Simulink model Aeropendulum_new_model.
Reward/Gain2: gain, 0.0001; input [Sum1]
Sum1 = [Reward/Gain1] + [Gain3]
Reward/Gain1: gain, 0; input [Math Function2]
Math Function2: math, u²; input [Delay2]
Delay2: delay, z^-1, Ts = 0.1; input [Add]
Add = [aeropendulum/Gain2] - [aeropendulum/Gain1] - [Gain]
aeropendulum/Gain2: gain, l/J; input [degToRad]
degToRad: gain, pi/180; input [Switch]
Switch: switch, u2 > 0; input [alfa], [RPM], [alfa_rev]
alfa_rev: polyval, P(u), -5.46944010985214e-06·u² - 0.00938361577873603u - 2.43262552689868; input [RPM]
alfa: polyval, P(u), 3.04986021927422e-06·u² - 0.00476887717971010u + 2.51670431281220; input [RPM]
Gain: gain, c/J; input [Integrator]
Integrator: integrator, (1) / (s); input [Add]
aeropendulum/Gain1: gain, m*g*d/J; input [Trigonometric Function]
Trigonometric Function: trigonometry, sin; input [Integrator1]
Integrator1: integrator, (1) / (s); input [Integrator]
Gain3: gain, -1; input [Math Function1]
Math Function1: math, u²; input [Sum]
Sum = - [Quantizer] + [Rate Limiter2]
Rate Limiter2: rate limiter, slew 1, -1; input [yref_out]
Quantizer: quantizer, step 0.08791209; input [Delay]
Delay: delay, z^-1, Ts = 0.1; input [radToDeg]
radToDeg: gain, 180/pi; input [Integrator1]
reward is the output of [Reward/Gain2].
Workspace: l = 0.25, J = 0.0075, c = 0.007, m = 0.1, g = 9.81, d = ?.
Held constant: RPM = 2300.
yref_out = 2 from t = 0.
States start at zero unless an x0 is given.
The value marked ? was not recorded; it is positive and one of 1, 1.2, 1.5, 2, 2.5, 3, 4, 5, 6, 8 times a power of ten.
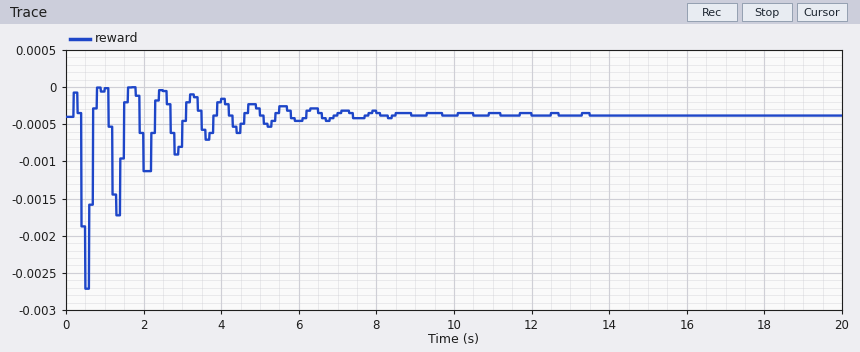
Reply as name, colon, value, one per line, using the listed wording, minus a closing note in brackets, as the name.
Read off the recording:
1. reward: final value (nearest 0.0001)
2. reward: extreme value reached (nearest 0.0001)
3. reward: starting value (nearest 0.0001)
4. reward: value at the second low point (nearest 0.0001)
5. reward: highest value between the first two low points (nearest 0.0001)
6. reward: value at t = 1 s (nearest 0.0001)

reward: final value: -0.0004
reward: extreme value reached: -0.0027
reward: starting value: -0.0004
reward: value at the second low point: -0.0017
reward: highest value between the first two low points: 0.0000
reward: value at t = 1 s: 0.0000
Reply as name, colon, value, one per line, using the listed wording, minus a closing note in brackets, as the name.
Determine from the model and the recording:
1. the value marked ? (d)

the value marked ?: 0.5
